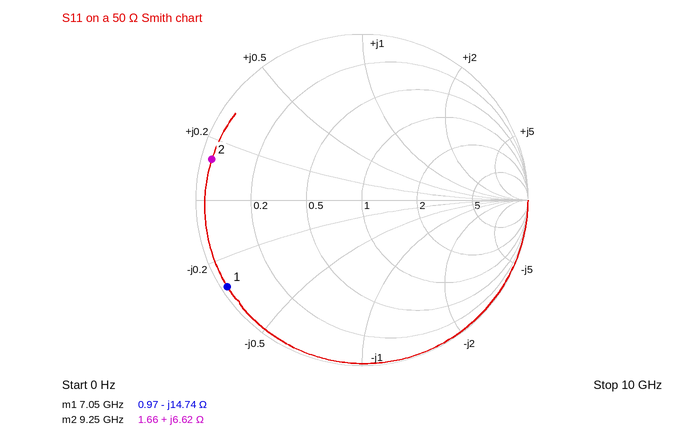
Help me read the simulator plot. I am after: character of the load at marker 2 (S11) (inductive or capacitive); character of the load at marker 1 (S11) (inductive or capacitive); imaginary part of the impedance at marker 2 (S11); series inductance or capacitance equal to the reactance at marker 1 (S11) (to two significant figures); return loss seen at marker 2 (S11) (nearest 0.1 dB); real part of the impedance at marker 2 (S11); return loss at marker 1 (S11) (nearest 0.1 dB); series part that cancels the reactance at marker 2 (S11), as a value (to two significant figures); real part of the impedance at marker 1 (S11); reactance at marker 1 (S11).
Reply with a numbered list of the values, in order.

1. inductive
2. capacitive
3. +6.62 Ω
4. 1.5 pF
5. 0.6 dB
6. 1.66 Ω
7. 0.3 dB
8. 2.6 pF
9. 0.97 Ω
10. -14.74 Ω
